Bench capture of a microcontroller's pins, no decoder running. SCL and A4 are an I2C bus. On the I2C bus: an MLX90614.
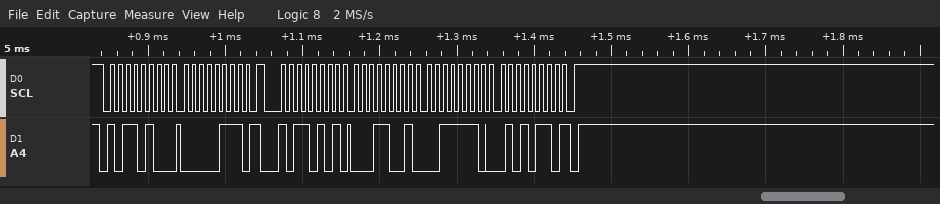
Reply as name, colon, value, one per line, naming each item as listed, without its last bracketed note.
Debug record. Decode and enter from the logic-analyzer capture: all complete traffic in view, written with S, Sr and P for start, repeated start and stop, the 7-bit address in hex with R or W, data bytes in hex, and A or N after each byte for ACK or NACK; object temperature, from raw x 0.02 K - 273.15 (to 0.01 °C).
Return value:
all complete traffic in view, written with S, Sr and P for start, repeated start and stop, the 7-bit address in hex with R or W, data bytes in hex, and A or N after each byte for ACK or NACK: S 5AW A 07 A Sr 5AR A 19 A 3E A 56 N P
object temperature, from raw x 0.02 K - 273.15: 44.79 °C
